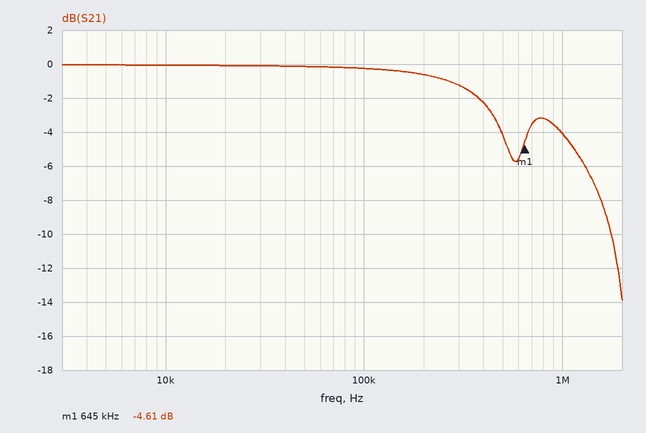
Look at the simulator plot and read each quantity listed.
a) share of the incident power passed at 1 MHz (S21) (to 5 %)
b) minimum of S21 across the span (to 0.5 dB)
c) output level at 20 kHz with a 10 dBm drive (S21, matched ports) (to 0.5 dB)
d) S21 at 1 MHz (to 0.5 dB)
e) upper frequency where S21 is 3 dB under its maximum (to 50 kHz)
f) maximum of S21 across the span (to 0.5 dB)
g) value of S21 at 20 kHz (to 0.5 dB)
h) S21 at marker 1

40 %
-14.0 dB
10.0 dBm
-4.0 dB
450 kHz
0.0 dB
0.0 dB
-4.61 dB
